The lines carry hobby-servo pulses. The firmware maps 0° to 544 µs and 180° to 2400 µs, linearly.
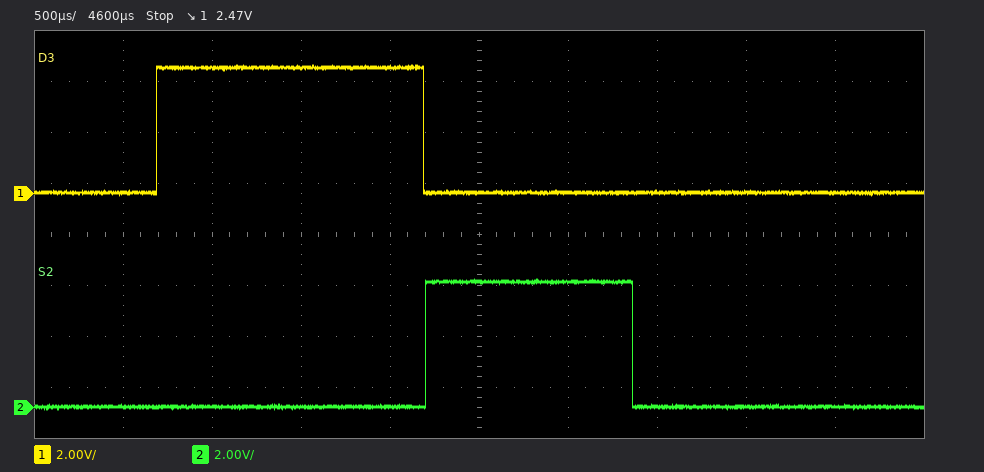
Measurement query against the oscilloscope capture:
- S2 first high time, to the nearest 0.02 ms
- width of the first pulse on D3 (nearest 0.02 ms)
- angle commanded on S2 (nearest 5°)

1.16 ms
1.50 ms
60°
